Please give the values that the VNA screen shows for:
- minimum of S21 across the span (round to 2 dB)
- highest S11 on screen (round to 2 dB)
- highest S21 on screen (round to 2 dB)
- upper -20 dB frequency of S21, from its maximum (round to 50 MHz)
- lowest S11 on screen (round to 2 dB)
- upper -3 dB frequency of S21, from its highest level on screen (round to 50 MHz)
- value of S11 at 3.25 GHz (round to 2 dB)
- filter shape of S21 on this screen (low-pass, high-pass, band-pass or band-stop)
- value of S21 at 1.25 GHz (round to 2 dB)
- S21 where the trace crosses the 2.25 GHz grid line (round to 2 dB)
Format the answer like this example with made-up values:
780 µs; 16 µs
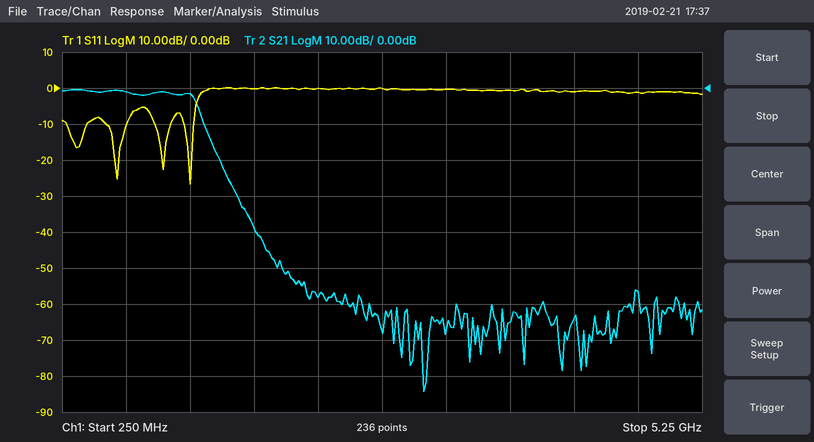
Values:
-84 dB; 0 dB; 0 dB; 1.50 GHz; -26 dB; 1.30 GHz; 0 dB; low-pass; -2 dB; -58 dB
